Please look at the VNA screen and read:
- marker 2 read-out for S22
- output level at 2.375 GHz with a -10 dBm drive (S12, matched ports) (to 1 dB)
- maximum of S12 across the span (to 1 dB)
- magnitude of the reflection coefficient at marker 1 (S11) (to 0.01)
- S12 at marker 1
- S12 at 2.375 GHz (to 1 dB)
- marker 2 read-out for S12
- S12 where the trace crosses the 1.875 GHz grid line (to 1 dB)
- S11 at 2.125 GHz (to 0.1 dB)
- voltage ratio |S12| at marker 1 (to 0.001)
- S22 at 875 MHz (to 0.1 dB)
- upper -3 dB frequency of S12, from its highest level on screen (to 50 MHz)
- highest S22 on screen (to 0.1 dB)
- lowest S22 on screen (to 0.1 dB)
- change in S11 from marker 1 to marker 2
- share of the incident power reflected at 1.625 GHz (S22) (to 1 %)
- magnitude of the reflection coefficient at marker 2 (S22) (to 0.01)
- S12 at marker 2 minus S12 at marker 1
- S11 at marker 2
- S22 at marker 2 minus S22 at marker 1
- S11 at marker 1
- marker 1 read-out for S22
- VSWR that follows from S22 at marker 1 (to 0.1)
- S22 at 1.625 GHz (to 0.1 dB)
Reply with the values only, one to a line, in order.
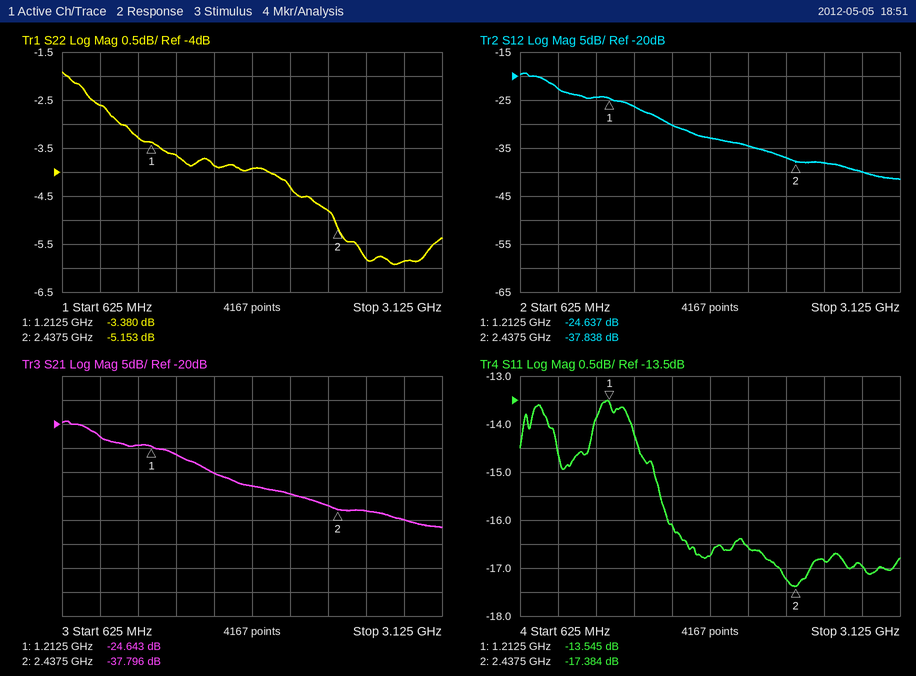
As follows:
-5.153 dB
-47 dBm
-19 dB
0.21
-24.637 dB
-37 dB
-37.838 dB
-33 dB
-16.6 dB
0.059
-2.6 dB
850 MHz
-1.9 dB
-5.9 dB
-3.839 dB
41 %
0.55
-13.201 dB
-17.384 dB
-1.773 dB
-13.545 dB
-3.380 dB
5.2
-3.9 dB
